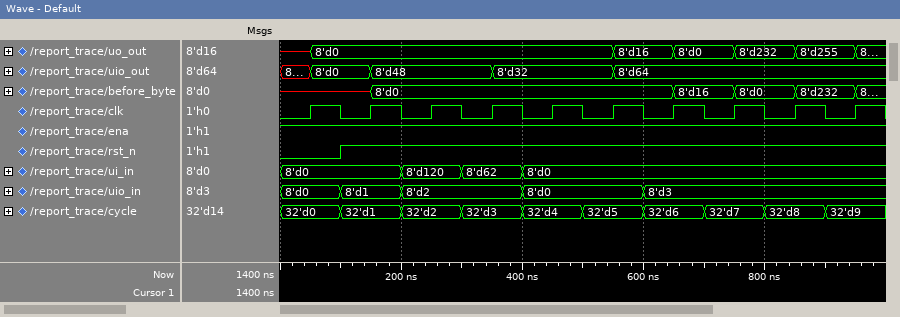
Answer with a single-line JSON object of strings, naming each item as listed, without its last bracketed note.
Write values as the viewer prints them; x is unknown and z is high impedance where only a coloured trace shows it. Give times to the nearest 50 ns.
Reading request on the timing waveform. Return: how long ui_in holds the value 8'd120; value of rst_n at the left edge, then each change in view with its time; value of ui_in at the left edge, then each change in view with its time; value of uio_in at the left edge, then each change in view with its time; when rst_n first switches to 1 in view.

{"how long ui_in holds the value 8'd120": "100 ns", "value of rst_n at the left edge, then each change in view with its time": "0, 1 at 100 ns", "value of ui_in at the left edge, then each change in view with its time": "8'd0, 8'd120 at 200 ns, 8'd62 at 300 ns, 8'd0 at 400 ns", "value of uio_in at the left edge, then each change in view with its time": "8'd0, 8'd1 at 100 ns, 8'd2 at 200 ns, 8'd0 at 400 ns, 8'd3 at 600 ns", "when rst_n first switches to 1 in view": "100 ns"}
